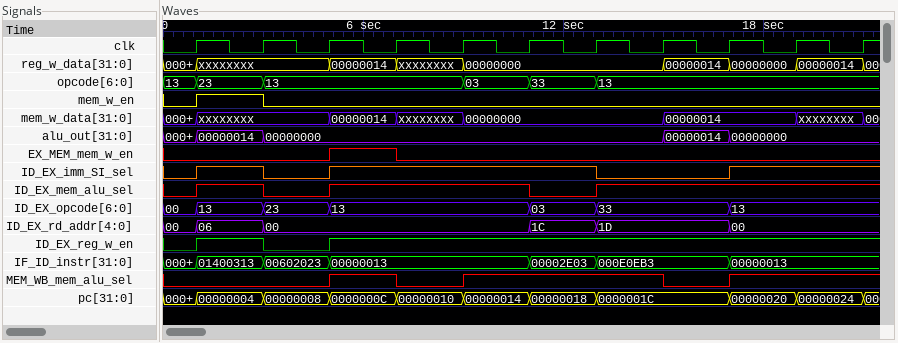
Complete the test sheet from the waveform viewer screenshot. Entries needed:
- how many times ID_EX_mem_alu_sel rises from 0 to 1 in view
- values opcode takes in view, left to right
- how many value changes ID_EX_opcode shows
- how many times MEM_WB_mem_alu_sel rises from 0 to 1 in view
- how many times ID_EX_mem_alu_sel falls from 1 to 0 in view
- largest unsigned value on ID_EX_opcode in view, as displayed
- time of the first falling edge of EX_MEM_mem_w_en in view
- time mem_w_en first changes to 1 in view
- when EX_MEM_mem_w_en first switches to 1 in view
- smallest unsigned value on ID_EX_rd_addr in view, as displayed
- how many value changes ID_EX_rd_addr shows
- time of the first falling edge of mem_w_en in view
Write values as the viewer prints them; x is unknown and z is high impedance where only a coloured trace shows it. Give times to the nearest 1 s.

3
13, 23, 13, 03, 33, 13
6
3
2
33
7 s
1 s
5 s
00
5
3 s
